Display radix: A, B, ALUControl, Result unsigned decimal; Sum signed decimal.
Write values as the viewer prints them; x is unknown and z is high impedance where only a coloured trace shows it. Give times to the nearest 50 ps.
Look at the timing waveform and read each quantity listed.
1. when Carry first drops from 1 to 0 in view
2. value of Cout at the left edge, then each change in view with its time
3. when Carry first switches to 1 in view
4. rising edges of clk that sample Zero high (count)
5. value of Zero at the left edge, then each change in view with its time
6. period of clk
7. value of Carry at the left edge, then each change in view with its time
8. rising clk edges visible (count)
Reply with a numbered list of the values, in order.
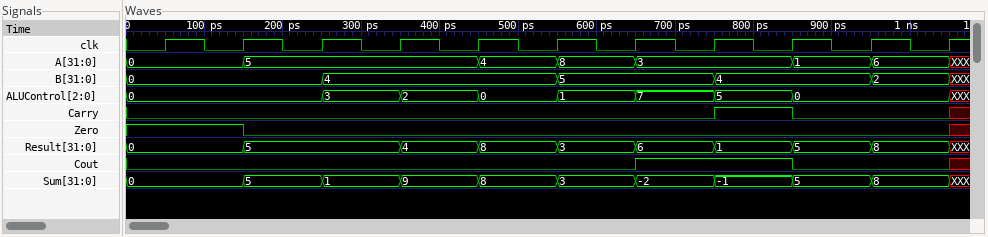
1. 850 ps
2. 0, 1 at 650 ps, 0 at 850 ps, x at 1050 ps
3. 750 ps
4. 2
5. 1, 0 at 150 ps, x at 1050 ps
6. 100 ps
7. 0, 1 at 750 ps, 0 at 850 ps, x at 1050 ps
8. 11
